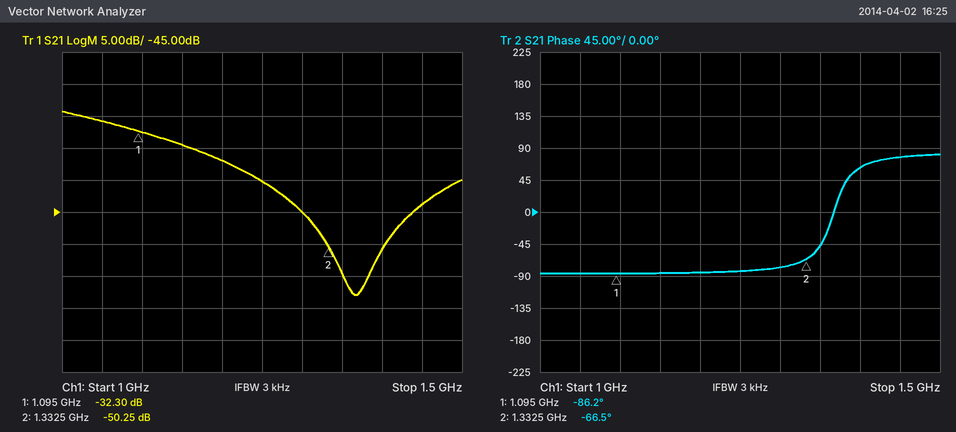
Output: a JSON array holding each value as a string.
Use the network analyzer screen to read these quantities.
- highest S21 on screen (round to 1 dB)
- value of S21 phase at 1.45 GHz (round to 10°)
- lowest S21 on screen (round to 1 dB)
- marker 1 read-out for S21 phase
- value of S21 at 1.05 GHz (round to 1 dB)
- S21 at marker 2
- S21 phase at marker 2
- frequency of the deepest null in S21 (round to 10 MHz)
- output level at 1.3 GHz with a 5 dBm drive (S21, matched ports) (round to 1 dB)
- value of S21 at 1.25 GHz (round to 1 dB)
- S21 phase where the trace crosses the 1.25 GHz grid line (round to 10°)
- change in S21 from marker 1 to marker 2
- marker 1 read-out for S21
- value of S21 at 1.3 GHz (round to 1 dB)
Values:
["-29 dB", "80°", "-58 dB", "-86.2°", "-31 dB", "-50.25 dB", "-66.5°", "1.37 GHz", "-40 dBm", "-40 dB", "-80°", "-17.95 dB", "-32.30 dB", "-45 dB"]
